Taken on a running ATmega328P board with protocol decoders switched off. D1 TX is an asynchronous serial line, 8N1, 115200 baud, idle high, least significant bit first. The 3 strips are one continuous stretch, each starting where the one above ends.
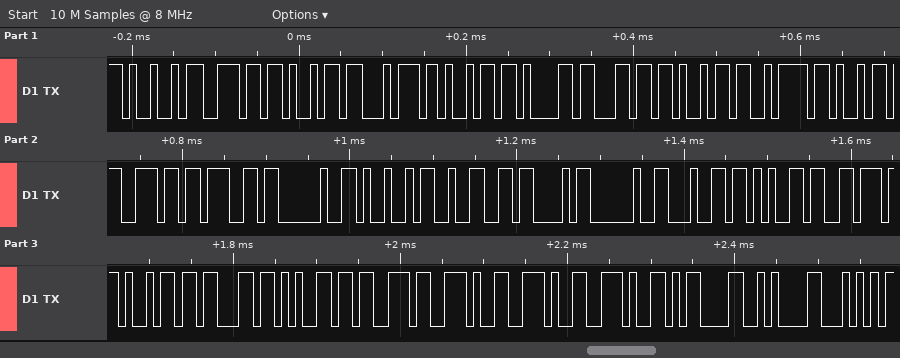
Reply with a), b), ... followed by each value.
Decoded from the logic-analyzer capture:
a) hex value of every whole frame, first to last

a) 49 6E 69 74 69 61 6C 69 7A 69 6E 67 20 49 32 43 20 64 65 76 69 63 65 73 2E 2E 2E 0D 0A 54
